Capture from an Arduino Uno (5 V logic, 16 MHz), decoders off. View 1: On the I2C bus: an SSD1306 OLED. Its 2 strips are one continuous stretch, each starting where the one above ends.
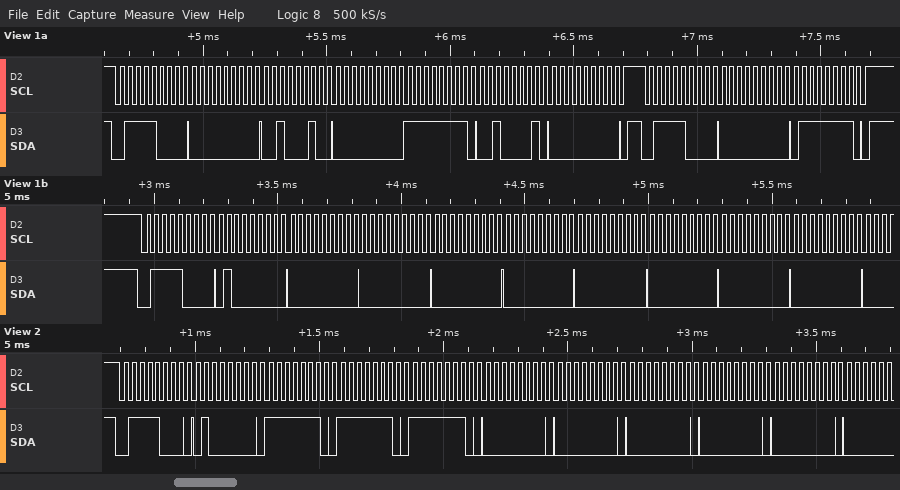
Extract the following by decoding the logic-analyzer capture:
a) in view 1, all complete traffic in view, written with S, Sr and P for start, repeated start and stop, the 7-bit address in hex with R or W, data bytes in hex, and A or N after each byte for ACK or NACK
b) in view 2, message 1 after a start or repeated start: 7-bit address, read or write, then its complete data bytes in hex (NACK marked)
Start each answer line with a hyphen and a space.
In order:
- S 3CW A 00 A 22 A 00 A FF A 21 A 00 A P S 3CW A 00 A 7F A P S 3CW A 40 A 00 A 00 A 00 A 00 A 00 A 00 A 00 A 00 A
- 0x3C write: 40 FE FE FE 00 00 00 00 00
